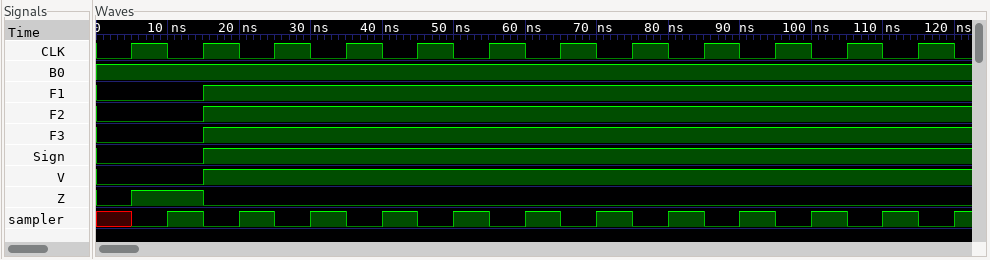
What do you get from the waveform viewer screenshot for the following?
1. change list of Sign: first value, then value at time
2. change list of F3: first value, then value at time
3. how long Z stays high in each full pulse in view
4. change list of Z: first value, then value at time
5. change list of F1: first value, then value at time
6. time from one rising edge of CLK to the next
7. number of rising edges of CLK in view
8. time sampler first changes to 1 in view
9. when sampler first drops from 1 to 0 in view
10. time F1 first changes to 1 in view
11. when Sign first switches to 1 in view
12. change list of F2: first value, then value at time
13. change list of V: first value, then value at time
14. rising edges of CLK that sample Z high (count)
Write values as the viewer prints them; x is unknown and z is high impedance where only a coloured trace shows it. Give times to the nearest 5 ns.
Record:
0, 1 at 15 ns
0, 1 at 15 ns
10 ns
0, 1 at 5 ns, 0 at 15 ns
0, 1 at 15 ns
10 ns
12
10 ns
15 ns
15 ns
15 ns
0, 1 at 15 ns
0, 1 at 15 ns
1
